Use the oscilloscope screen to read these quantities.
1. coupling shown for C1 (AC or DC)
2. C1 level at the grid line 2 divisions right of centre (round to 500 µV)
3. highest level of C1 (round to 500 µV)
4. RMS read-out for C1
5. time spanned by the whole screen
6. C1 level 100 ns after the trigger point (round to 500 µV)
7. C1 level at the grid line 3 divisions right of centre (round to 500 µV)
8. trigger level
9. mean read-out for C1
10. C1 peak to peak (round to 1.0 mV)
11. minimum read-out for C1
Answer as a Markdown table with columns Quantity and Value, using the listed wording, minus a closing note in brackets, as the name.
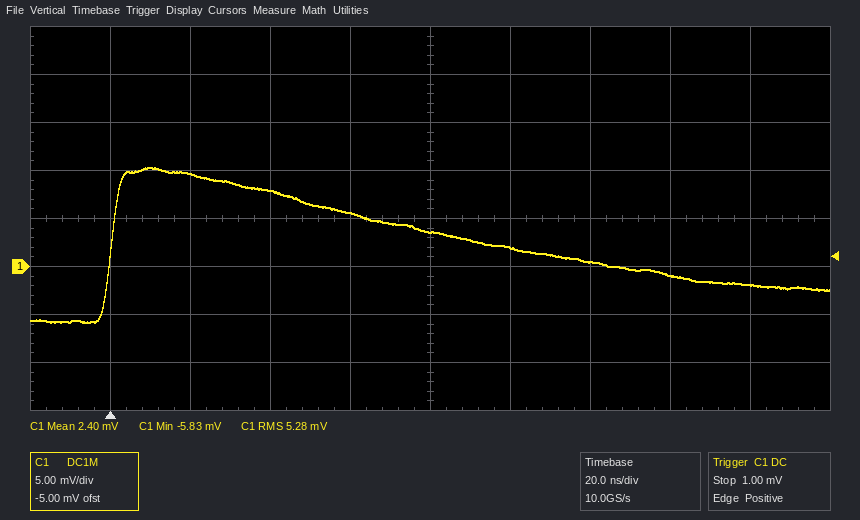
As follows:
| Quantity | Value |
|---|---|
| coupling shown for C1 | DC |
| C1 level at the grid line 2 divisions right of centre | 500 µV |
| highest level of C1 | 10.5 mV |
| RMS read-out for C1 | 5.28 mV |
| time spanned by the whole screen | 200 ns |
| C1 level 100 ns after the trigger point | 2.0 mV |
| C1 level at the grid line 3 divisions right of centre | -1.0 mV |
| trigger level | 1.00 mV |
| mean read-out for C1 | 2.40 mV |
| C1 peak to peak | 16.0 mV |
| minimum read-out for C1 | -5.83 mV |
